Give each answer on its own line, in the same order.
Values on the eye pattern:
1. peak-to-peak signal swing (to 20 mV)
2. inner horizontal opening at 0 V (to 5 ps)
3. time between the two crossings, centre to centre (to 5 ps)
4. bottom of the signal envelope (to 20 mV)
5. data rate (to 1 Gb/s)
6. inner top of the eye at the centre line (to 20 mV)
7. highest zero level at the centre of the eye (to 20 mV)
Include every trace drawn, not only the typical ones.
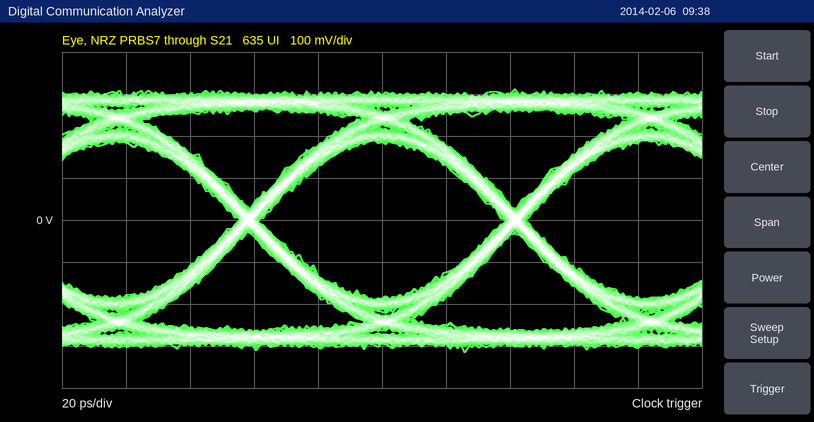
620 mV
75 ps
85 ps
-320 mV
12 Gb/s
180 mV
-180 mV
